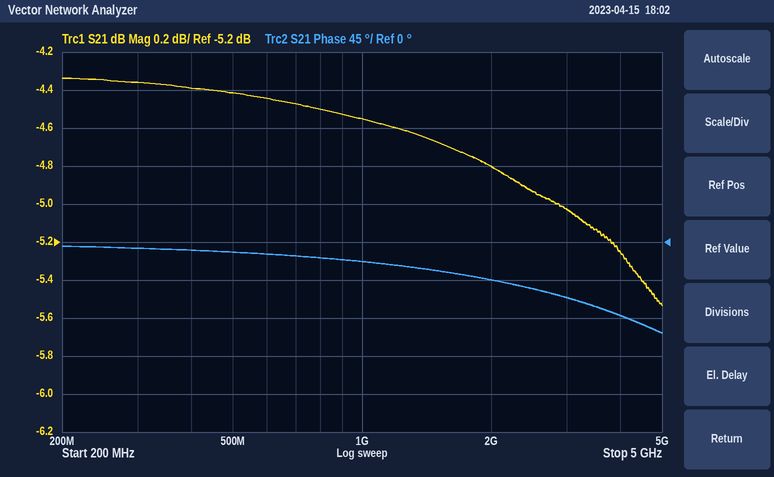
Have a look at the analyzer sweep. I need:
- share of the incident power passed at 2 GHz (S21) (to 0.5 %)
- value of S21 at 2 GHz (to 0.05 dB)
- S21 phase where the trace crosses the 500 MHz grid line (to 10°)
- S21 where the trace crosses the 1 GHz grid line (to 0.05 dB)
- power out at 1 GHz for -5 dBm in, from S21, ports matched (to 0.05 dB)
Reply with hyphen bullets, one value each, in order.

- 33.0 %
- -4.80 dB
- -10°
- -4.55 dB
- -9.55 dBm
